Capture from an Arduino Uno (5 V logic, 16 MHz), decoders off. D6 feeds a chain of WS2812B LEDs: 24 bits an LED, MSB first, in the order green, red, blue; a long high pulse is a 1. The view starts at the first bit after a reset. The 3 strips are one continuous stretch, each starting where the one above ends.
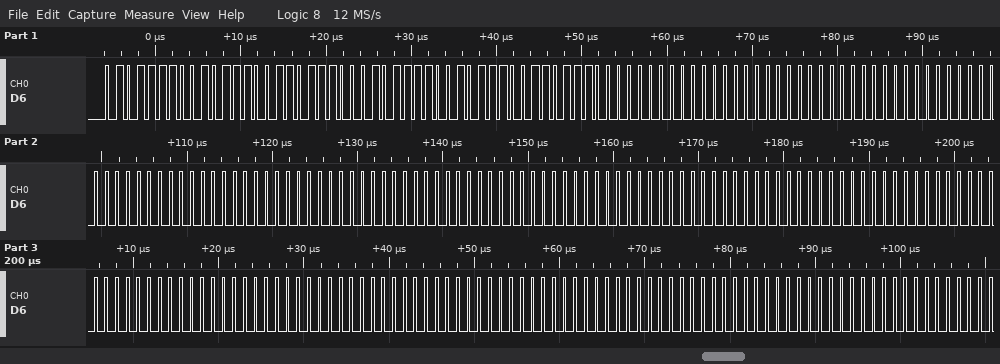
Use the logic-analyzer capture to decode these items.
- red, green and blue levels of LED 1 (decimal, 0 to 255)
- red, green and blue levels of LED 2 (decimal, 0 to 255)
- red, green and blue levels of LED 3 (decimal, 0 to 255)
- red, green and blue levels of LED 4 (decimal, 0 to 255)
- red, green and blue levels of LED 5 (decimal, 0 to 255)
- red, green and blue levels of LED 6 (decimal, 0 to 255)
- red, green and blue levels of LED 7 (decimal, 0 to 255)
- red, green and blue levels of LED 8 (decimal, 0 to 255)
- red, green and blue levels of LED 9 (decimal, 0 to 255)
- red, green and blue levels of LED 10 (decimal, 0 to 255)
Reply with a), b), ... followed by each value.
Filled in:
a) 92, 94, 220
b) 92, 94, 220
c) 0, 0, 0
d) 0, 0, 0
e) 0, 0, 0
f) 0, 0, 0
g) 0, 0, 0
h) 0, 0, 0
i) 0, 0, 0
j) 0, 0, 0
